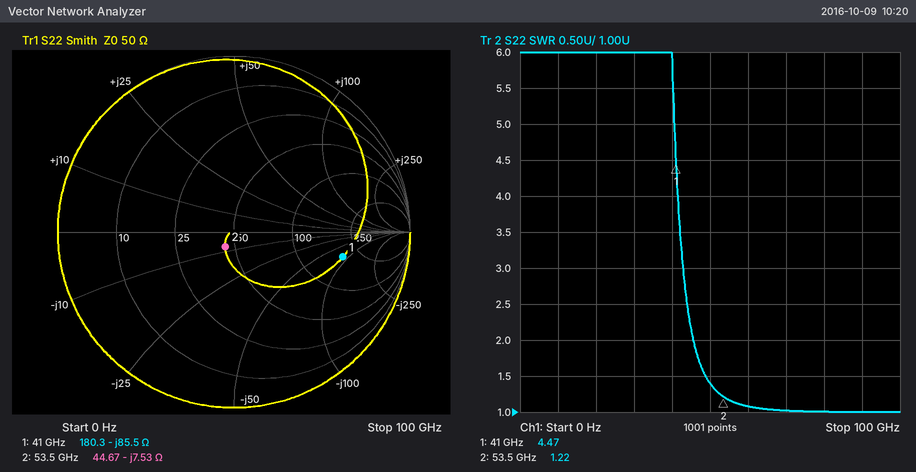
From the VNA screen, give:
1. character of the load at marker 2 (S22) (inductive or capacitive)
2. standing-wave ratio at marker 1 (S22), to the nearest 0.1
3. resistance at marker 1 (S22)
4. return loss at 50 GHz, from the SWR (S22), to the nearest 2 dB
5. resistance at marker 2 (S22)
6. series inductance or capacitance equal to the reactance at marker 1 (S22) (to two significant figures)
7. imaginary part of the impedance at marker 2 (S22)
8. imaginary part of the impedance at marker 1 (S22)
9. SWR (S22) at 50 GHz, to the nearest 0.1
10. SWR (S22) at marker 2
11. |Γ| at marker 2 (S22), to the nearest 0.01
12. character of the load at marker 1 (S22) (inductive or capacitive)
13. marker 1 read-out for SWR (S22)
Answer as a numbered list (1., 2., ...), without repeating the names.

1. capacitive
2. 4.5
3. 180.3 Ω
4. 16 dB
5. 44.67 Ω
6. 45 fF
7. -7.53 Ω
8. -85.5 Ω
9. 1.4
10. 1.22
11. 0.10
12. capacitive
13. 4.47
